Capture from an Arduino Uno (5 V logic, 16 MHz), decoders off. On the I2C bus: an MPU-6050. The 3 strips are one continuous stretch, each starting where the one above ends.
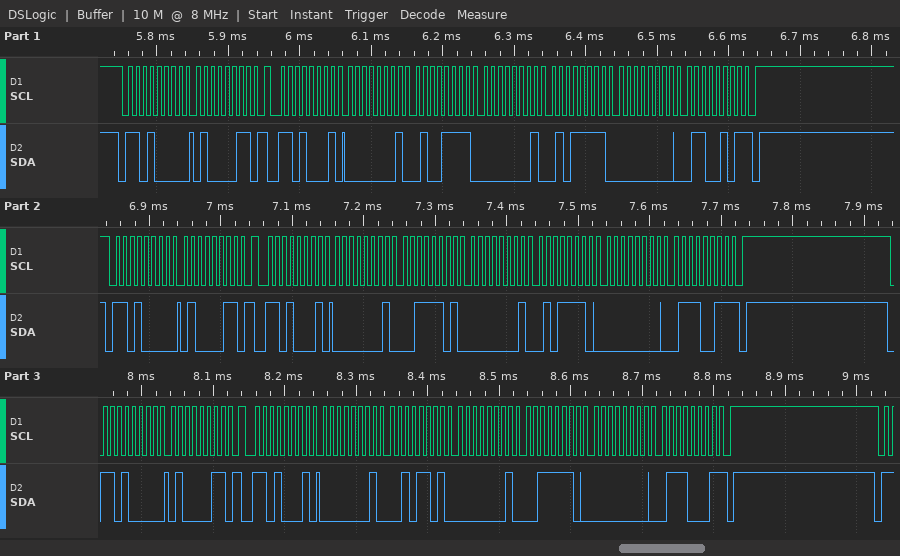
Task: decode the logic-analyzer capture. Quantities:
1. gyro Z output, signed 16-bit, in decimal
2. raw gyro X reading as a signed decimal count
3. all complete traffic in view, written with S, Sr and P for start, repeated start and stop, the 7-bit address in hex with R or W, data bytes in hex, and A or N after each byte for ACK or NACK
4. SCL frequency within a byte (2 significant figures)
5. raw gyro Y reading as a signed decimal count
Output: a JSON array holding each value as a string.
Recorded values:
["101", "335", "S 68W A 43 A Sr 68R A 01 A 4F A 01 A 5F A 00 A 65 N P S 68W A 43 A Sr 68R A 01 A 3D A 01 A 5E A 00 A 73 N P S 68W A 43 A Sr 68R A 01 A 2D A 01 A 3E A 00 A 71 N P", "100 kHz", "351"]
